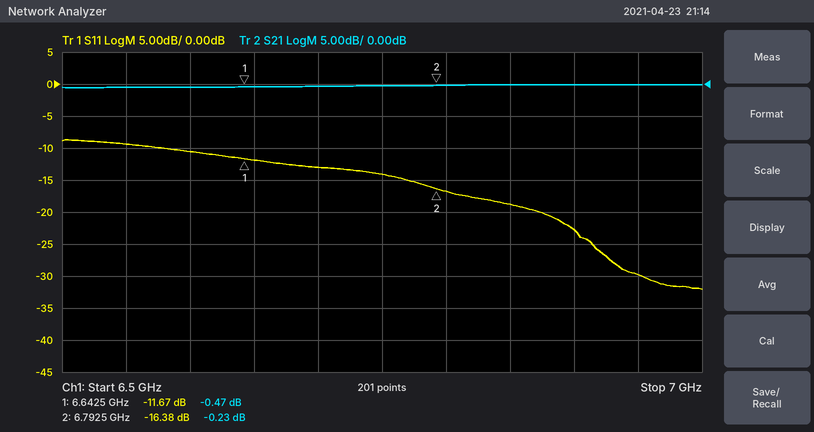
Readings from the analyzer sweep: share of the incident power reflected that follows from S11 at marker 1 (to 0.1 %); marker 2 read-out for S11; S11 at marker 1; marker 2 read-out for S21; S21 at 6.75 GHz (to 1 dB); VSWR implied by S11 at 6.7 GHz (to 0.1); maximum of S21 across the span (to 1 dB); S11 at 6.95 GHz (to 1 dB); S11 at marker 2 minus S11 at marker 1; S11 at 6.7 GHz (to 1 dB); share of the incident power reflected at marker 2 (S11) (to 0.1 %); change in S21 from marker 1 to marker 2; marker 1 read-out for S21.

6.8 %
-16.38 dB
-11.67 dB
-0.23 dB
0 dB
1.6
0 dB
-30 dB
-4.71 dB
-13 dB
2.3 %
0.24 dB
-0.47 dB
